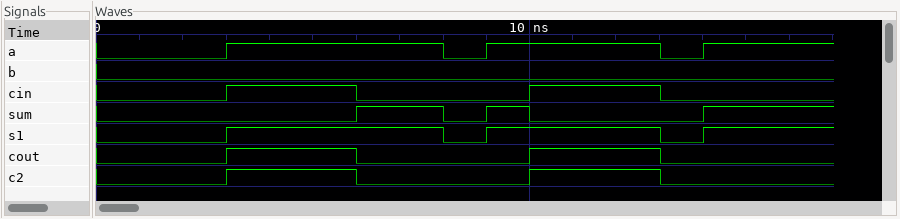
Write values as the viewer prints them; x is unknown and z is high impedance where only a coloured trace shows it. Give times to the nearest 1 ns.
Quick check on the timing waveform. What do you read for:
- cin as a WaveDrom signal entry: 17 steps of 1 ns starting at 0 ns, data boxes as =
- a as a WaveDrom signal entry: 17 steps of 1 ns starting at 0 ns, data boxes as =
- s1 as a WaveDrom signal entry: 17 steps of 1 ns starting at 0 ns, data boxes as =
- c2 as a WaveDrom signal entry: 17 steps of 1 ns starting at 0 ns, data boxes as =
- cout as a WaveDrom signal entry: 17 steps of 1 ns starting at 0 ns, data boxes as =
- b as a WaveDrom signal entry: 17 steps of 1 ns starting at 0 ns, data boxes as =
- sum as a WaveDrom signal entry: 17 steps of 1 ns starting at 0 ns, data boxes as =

{name: 'cin', wave: '0..1..0...1..0...'}
{name: 'a', wave: '0..1....01...01..'}
{name: 's1', wave: '0..1....01...01..'}
{name: 'c2', wave: '0..1..0...1..0...'}
{name: 'cout', wave: '0..1..0...1..0...'}
{name: 'b', wave: '0................'}
{name: 'sum', wave: '0.....1.010...1..'}
